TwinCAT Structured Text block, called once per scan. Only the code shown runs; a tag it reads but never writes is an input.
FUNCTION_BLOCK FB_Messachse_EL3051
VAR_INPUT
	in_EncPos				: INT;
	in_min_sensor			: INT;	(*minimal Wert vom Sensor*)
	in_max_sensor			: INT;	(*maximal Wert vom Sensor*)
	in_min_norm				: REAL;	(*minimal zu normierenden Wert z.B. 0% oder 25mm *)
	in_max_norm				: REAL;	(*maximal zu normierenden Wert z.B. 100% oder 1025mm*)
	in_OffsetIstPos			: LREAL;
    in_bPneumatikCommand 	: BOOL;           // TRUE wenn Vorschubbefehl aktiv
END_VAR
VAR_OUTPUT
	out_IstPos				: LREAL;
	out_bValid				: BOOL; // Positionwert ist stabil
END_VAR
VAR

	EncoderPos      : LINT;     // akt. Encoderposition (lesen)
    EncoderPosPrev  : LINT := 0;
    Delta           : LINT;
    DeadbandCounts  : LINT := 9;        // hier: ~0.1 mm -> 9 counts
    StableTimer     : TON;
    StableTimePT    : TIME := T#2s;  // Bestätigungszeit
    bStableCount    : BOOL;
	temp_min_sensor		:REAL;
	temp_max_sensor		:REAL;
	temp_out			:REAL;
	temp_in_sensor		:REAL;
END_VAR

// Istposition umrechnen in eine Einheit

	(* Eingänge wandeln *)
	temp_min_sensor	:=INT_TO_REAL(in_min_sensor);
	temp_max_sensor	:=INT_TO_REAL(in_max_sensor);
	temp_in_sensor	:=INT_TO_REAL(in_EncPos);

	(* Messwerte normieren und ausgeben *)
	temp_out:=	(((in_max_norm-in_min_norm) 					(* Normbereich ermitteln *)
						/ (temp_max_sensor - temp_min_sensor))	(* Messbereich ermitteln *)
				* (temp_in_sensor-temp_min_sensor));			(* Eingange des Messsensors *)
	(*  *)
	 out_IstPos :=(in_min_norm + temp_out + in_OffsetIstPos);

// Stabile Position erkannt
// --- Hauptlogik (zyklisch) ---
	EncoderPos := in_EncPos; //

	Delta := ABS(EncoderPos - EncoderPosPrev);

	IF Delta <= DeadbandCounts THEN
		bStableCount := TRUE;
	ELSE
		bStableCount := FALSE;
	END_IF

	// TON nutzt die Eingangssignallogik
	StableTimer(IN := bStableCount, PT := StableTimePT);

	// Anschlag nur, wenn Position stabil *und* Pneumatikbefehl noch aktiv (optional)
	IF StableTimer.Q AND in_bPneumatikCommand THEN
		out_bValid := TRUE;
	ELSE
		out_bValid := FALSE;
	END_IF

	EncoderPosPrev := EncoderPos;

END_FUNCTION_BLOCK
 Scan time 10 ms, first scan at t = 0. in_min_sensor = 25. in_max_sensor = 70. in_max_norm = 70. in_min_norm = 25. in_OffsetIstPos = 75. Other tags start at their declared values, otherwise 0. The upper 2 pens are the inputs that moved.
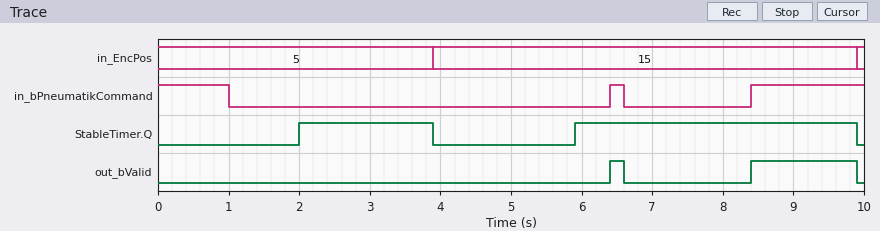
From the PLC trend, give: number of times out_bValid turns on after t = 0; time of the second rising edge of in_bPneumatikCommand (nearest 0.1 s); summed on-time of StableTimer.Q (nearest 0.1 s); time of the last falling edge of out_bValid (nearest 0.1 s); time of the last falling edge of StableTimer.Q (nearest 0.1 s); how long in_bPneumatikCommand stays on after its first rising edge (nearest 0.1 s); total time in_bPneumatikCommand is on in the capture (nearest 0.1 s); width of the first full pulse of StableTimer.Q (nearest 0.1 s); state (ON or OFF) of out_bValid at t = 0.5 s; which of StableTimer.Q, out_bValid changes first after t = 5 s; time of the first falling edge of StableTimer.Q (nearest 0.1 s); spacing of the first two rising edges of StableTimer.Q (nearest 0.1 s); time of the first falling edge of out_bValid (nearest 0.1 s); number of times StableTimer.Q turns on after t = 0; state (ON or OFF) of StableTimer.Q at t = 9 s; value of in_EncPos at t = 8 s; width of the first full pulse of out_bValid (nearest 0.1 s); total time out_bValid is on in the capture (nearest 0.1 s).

2
8.4 s
5.9 s
9.9 s
9.9 s
0.2 s
2.8 s
1.9 s
OFF
StableTimer.Q
3.9 s
3.9 s
6.6 s
2
ON
15
0.2 s
1.7 s
